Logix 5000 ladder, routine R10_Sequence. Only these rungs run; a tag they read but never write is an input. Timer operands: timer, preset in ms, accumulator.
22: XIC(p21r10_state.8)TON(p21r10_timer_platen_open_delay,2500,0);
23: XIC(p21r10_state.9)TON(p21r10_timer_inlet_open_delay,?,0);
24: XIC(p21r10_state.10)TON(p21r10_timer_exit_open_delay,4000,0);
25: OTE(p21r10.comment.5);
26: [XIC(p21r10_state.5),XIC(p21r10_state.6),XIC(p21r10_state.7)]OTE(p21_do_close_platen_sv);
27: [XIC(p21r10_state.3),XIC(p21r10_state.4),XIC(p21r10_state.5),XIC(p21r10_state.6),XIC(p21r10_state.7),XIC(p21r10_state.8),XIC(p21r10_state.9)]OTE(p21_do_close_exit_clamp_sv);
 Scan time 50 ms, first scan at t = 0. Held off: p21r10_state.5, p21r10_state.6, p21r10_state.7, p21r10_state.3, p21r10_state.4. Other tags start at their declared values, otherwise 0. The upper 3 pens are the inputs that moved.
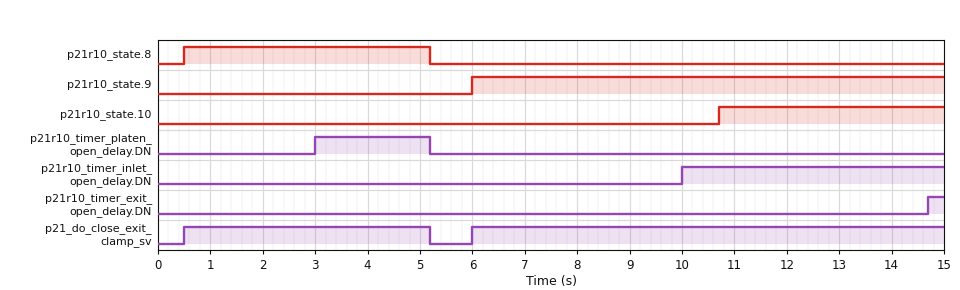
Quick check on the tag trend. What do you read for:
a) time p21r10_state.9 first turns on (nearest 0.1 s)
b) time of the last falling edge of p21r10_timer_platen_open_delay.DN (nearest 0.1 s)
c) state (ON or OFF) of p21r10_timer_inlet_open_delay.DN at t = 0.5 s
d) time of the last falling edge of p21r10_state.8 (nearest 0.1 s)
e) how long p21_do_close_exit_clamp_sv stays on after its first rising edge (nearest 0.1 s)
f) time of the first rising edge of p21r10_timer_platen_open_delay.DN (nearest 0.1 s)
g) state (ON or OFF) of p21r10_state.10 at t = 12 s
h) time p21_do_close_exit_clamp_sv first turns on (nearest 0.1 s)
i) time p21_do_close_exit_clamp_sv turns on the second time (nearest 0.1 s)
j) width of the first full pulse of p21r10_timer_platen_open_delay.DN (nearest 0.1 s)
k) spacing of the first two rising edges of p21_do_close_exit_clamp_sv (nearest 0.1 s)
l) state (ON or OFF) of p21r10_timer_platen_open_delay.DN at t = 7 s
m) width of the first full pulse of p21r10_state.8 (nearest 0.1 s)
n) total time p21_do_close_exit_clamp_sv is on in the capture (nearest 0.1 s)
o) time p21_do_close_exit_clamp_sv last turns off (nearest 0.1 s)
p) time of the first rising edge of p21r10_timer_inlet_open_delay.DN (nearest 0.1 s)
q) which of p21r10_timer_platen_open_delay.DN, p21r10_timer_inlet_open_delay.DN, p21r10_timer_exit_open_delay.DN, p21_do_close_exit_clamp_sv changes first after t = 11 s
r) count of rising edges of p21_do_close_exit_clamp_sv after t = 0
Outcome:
6.0 s
5.2 s
OFF
5.2 s
4.7 s
3.0 s
ON
0.5 s
6.0 s
2.2 s
5.5 s
OFF
4.7 s
13.7 s
5.2 s
10.0 s
p21r10_timer_exit_open_delay.DN
2
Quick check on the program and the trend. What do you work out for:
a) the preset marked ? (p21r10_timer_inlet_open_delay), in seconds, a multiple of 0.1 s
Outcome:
4.0 s
